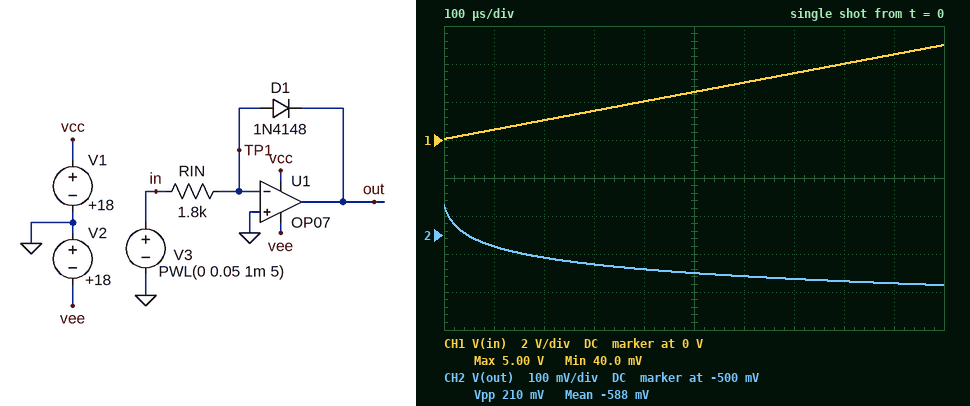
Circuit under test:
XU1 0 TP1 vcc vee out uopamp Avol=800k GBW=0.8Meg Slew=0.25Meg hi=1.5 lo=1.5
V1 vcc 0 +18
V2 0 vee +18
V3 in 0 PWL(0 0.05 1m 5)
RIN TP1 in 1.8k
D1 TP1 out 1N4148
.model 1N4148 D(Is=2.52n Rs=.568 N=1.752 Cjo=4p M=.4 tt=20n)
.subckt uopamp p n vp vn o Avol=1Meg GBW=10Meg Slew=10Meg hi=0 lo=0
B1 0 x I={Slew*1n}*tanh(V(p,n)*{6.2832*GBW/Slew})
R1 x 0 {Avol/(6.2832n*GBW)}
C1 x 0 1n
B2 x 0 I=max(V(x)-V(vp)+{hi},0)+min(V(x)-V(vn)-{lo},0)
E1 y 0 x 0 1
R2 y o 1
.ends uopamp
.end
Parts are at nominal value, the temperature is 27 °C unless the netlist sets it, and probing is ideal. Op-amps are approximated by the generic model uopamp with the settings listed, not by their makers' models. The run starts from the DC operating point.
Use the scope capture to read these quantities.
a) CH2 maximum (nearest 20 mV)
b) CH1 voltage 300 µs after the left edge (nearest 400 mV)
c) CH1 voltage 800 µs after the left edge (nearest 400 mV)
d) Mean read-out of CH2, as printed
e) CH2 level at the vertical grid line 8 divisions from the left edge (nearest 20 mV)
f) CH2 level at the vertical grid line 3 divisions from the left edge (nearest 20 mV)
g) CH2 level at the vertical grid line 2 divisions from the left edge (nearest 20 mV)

-420 mV
1.6 V
4.0 V
-588 mV
-620 mV
-580 mV
-560 mV
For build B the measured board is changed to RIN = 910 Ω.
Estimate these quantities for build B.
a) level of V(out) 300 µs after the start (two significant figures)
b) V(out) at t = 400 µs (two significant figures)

-610 mV
-620 mV
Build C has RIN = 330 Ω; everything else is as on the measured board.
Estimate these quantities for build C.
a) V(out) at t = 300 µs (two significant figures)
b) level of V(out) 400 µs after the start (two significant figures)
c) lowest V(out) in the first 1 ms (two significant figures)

-660 mV
-670 mV
-720 mV
